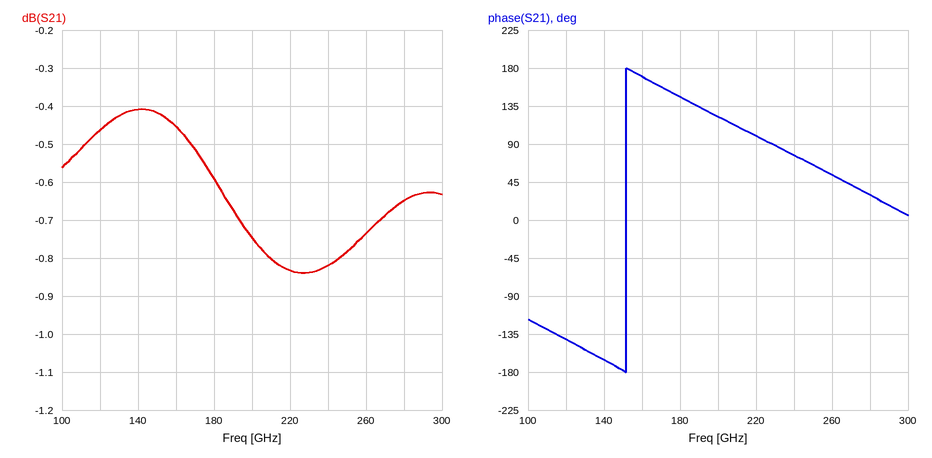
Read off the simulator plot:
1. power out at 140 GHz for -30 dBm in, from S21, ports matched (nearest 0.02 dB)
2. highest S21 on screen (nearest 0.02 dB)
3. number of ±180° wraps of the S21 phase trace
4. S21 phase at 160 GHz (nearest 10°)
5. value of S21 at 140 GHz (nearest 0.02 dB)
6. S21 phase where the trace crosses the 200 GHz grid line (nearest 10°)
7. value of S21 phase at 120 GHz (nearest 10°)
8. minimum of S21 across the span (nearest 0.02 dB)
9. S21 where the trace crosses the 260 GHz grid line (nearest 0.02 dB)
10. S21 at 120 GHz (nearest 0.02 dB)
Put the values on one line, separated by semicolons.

-30.40 dBm; -0.40 dB; 1; 170°; -0.40 dB; 120°; -140°; -0.84 dB; -0.74 dB; -0.46 dB
